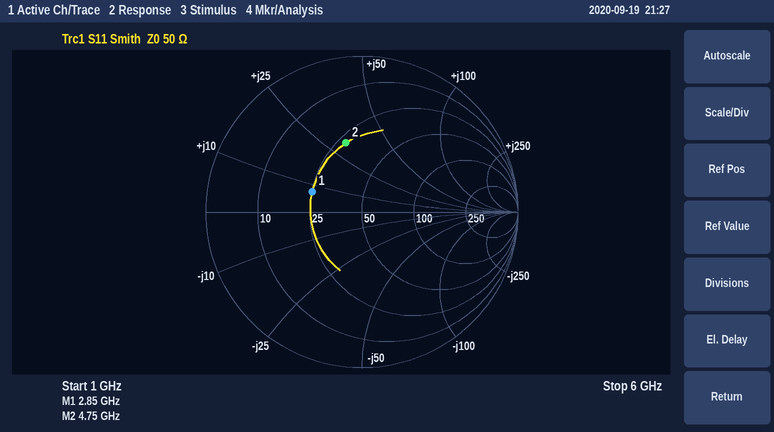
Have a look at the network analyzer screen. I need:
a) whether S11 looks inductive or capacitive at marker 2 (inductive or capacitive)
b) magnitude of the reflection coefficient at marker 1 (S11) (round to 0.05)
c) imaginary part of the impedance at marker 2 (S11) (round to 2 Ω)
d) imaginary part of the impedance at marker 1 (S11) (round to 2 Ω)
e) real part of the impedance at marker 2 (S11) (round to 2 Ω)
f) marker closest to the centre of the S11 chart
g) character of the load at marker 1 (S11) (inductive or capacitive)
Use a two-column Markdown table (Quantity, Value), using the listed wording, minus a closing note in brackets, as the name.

| Quantity | Value |
|---|---|
| whether S11 looks inductive or capacitive at marker 2 | inductive |
| magnitude of the reflection coefficient at marker 1 (S11) | 0.35 |
| imaginary part of the impedance at marker 2 (S11) | +32 Ω |
| imaginary part of the impedance at marker 1 (S11) | +8 Ω |
| real part of the impedance at marker 2 (S11) | 28 Ω |
| marker closest to the centre of the S11 chart | marker 1 |
| character of the load at marker 1 (S11) | inductive |
